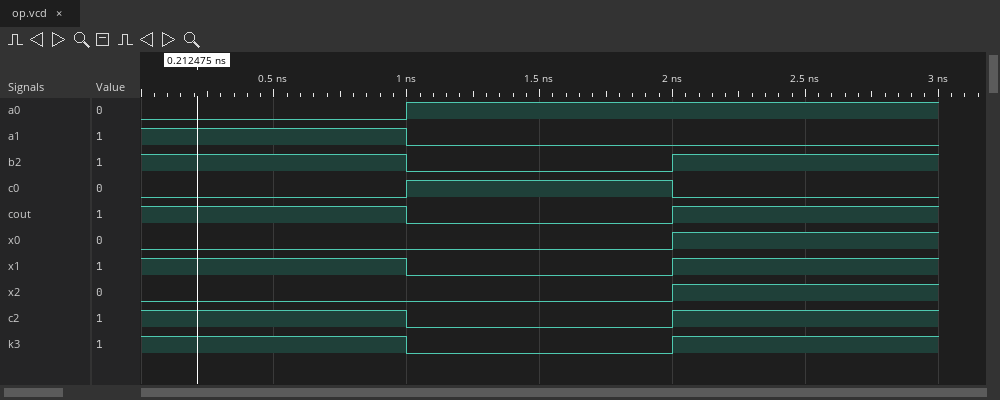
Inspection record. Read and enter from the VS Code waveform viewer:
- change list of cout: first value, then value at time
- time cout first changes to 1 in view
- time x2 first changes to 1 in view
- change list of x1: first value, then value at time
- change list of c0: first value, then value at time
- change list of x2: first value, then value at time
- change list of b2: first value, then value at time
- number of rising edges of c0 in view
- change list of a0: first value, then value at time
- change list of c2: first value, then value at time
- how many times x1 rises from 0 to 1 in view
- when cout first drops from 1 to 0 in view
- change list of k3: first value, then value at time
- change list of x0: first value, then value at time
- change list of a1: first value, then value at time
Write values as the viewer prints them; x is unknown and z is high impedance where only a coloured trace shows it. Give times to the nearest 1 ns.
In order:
1, 0 at 1 ns, 1 at 2 ns
2 ns
2 ns
1, 0 at 1 ns, 1 at 2 ns
0, 1 at 1 ns, 0 at 2 ns
0, 1 at 2 ns
1, 0 at 1 ns, 1 at 2 ns
1
0, 1 at 1 ns
1, 0 at 1 ns, 1 at 2 ns
1
1 ns
1, 0 at 1 ns, 1 at 2 ns
0, 1 at 2 ns
1, 0 at 1 ns
